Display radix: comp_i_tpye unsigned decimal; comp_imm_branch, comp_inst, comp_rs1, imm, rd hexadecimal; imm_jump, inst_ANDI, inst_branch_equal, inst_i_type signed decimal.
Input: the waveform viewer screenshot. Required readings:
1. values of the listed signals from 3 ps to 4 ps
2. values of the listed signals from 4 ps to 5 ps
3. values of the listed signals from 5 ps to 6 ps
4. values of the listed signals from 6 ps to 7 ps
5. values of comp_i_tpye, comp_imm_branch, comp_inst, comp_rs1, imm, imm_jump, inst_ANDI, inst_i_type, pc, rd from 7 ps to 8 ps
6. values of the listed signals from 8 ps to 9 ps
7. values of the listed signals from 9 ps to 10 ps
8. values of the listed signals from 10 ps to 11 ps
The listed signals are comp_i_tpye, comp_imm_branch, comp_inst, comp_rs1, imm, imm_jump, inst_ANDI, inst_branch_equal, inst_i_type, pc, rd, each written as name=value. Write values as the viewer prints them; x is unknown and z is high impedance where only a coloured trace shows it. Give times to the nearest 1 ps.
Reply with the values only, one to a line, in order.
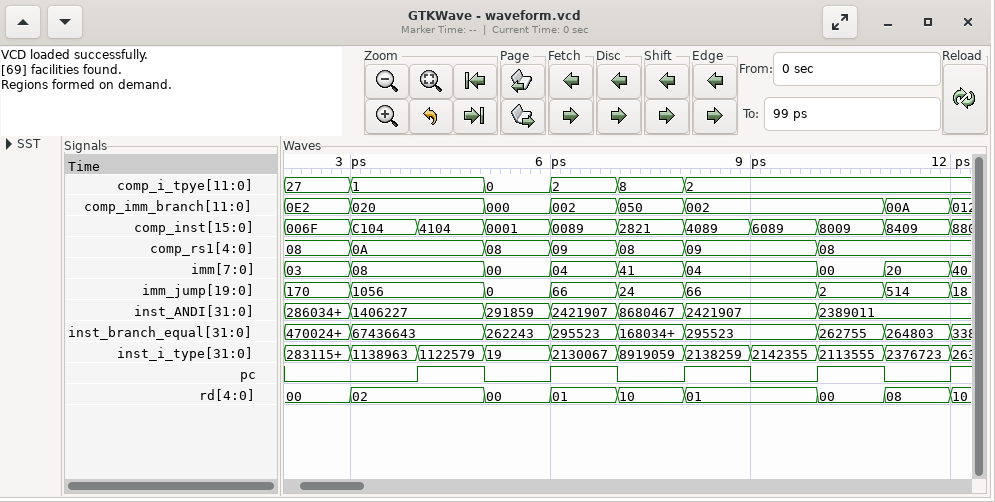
comp_i_tpye=1, comp_imm_branch=020, comp_inst=C104, comp_rs1=0A, imm=08, imm_jump=1056, inst_ANDI=1406227, inst_branch_equal=67436643, inst_i_type=1138963, pc=0, rd=02
comp_i_tpye=1, comp_imm_branch=020, comp_inst=4104, comp_rs1=0A, imm=08, imm_jump=1056, inst_ANDI=1406227, inst_branch_equal=67436643, inst_i_type=1122579, pc=1, rd=02
comp_i_tpye=0, comp_imm_branch=000, comp_inst=0001, comp_rs1=08, imm=00, imm_jump=0, inst_ANDI=291859, inst_branch_equal=262243, inst_i_type=19, pc=0, rd=00
comp_i_tpye=2, comp_imm_branch=002, comp_inst=0089, comp_rs1=09, imm=04, imm_jump=66, inst_ANDI=2421907, inst_branch_equal=295523, inst_i_type=2130067, pc=1, rd=01
comp_i_tpye=8, comp_imm_branch=050, comp_inst=2821, comp_rs1=08, imm=41, imm_jump=24, inst_ANDI=8680467, inst_i_type=8919059, pc=0, rd=10
comp_i_tpye=2, comp_imm_branch=002, comp_inst=4089, comp_rs1=09, imm=04, imm_jump=66, inst_ANDI=2421907, inst_branch_equal=295523, inst_i_type=2138259, pc=1, rd=01
comp_i_tpye=2, comp_imm_branch=002, comp_inst=6089, comp_rs1=09, imm=04, imm_jump=66, inst_ANDI=2421907, inst_branch_equal=295523, inst_i_type=2142355, pc=0, rd=01
comp_i_tpye=2, comp_imm_branch=002, comp_inst=8009, comp_rs1=08, imm=00, imm_jump=2, inst_ANDI=2389011, inst_branch_equal=262755, inst_i_type=2113555, pc=1, rd=00
